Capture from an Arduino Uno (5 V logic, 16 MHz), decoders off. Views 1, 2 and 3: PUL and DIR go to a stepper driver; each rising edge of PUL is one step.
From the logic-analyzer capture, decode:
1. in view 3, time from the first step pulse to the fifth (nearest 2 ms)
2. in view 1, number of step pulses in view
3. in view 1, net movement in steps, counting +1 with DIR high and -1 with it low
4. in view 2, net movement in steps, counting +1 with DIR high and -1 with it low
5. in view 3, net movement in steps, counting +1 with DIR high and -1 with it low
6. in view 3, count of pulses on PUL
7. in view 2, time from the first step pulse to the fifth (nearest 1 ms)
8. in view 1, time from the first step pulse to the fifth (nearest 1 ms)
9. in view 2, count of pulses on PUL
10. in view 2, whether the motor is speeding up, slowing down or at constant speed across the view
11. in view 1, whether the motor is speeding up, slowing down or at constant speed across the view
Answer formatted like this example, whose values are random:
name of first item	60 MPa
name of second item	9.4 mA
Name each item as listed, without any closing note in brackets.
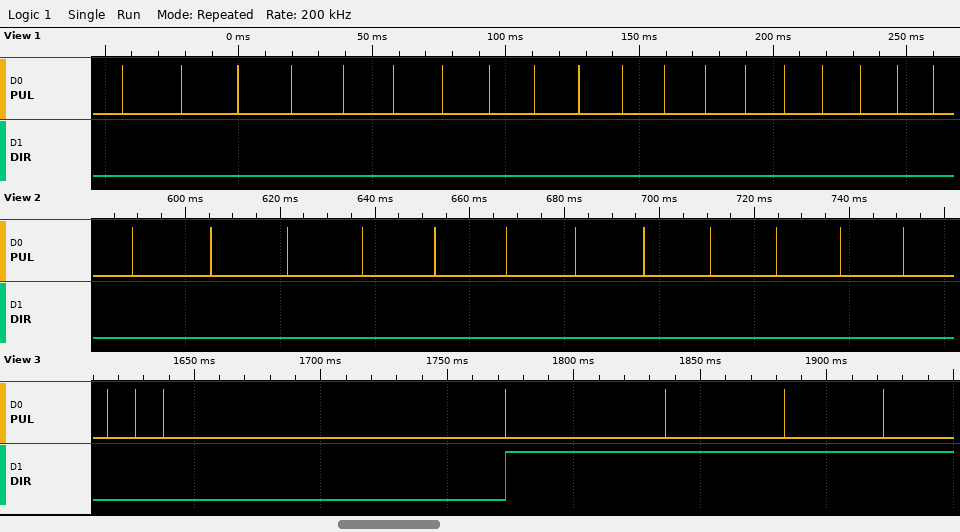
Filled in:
in view 3, time from the first step pulse to the fifth	220 ms
in view 1, number of step pulses in view	19
in view 1, net movement in steps, counting +1 with DIR high and -1 with it low	-19
in view 2, net movement in steps, counting +1 with DIR high and -1 with it low	-12
in view 3, net movement in steps, counting +1 with DIR high and -1 with it low	+1
in view 3, count of pulses on PUL	7
in view 2, time from the first step pulse to the fifth	64 ms
in view 1, time from the first step pulse to the fifth	83 ms
in view 2, count of pulses on PUL	12
in view 2, whether the motor is speeding up, slowing down or at constant speed across the view	speeding up
in view 1, whether the motor is speeding up, slowing down or at constant speed across the view	speeding up
